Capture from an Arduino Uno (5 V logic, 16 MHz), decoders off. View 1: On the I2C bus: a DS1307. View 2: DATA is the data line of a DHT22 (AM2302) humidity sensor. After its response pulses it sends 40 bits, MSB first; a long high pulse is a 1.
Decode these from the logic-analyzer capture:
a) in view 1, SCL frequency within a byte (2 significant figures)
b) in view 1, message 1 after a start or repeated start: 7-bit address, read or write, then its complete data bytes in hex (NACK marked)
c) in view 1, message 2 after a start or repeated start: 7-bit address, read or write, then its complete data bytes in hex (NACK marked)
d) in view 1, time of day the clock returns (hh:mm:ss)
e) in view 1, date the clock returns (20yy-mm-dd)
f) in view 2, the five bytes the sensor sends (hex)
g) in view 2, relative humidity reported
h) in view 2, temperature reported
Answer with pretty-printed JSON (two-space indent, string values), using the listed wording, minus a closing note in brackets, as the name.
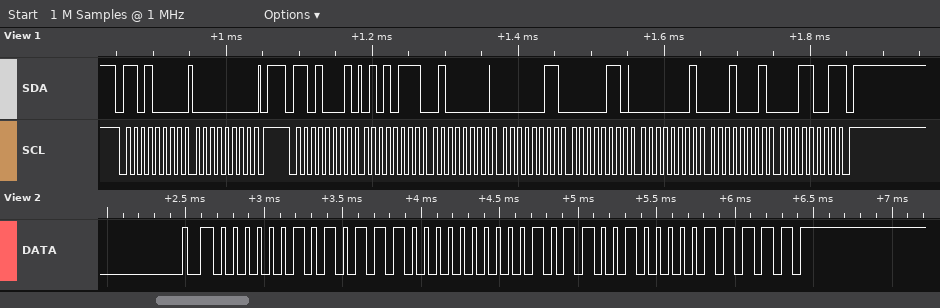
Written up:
{
  "in view 1, SCL frequency within a byte": "100 kHz",
  "in view 1, message 1 after a start or repeated start: 7-bit address, read or write, then its complete data bytes in hex": "0x68 write: 00",
  "in view 1, message 2 after a start or repeated start: 7-bit address, read or write, then its complete data bytes in hex": "0x68 read: 57 40 03 06 01 11 19 NACK",
  "in view 1, time of day the clock returns": "03:40:57",
  "in view 1, date the clock returns": "2019-11-01",
  "in view 2, the five bytes the sensor sends": "02 B8 01 64 1F",
  "in view 2, relative humidity reported": "69.6 %",
  "in view 2, temperature reported": "35.6 °C"
}
